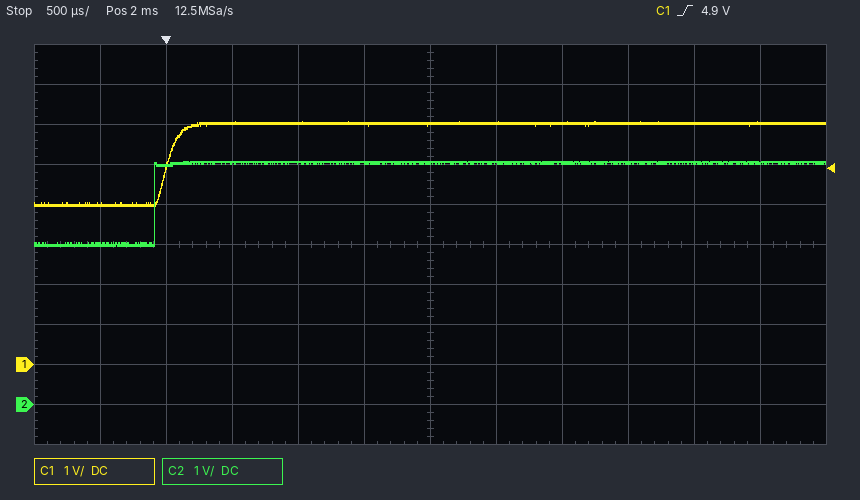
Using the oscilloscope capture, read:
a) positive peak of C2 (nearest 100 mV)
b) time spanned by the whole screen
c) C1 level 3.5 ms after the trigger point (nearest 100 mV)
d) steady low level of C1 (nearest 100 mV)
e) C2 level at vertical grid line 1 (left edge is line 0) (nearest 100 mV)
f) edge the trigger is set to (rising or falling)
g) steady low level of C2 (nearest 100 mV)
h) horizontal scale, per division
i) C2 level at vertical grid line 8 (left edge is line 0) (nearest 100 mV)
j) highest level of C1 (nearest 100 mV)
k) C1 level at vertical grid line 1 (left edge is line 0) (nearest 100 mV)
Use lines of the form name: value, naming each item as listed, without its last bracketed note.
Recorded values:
positive peak of C2: 6.1 V
time spanned by the whole screen: 6 ms
C1 level 3.5 ms after the trigger point: 6.0 V
steady low level of C1: 4.0 V
C2 level at vertical grid line 1 (left edge is line 0): 4.0 V
edge the trigger is set to: rising
steady low level of C2: 4.0 V
horizontal scale, per division: 500 µs
C2 level at vertical grid line 8 (left edge is line 0): 6.0 V
highest level of C1: 6.1 V
C1 level at vertical grid line 1 (left edge is line 0): 4.0 V
